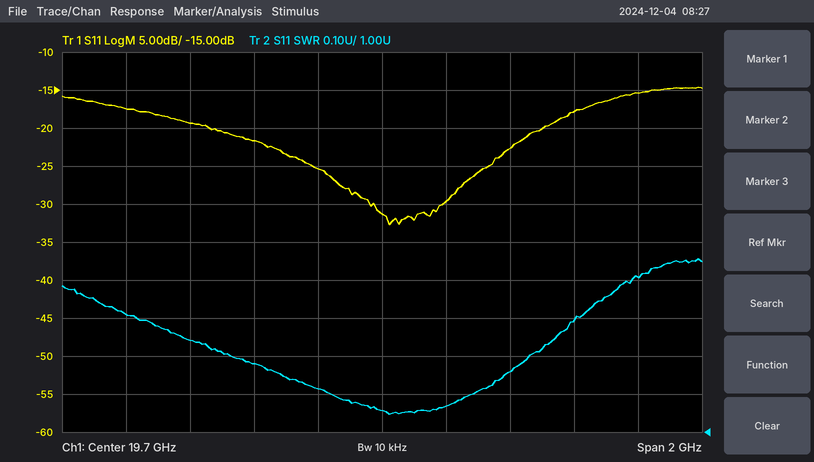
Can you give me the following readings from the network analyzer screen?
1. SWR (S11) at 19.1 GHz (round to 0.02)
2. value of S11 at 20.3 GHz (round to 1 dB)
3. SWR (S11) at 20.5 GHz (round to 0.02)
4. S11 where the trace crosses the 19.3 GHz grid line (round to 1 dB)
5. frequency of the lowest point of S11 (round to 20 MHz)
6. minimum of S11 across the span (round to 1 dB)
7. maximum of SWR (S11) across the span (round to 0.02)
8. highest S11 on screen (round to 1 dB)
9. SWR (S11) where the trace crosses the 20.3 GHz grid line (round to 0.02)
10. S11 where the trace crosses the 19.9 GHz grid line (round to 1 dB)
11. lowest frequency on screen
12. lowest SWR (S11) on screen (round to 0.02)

1.24
-18 dB
1.40
-22 dB
19.72 GHz
-33 dB
1.46
-15 dB
1.30
-30 dB
18.7 GHz
1.04
